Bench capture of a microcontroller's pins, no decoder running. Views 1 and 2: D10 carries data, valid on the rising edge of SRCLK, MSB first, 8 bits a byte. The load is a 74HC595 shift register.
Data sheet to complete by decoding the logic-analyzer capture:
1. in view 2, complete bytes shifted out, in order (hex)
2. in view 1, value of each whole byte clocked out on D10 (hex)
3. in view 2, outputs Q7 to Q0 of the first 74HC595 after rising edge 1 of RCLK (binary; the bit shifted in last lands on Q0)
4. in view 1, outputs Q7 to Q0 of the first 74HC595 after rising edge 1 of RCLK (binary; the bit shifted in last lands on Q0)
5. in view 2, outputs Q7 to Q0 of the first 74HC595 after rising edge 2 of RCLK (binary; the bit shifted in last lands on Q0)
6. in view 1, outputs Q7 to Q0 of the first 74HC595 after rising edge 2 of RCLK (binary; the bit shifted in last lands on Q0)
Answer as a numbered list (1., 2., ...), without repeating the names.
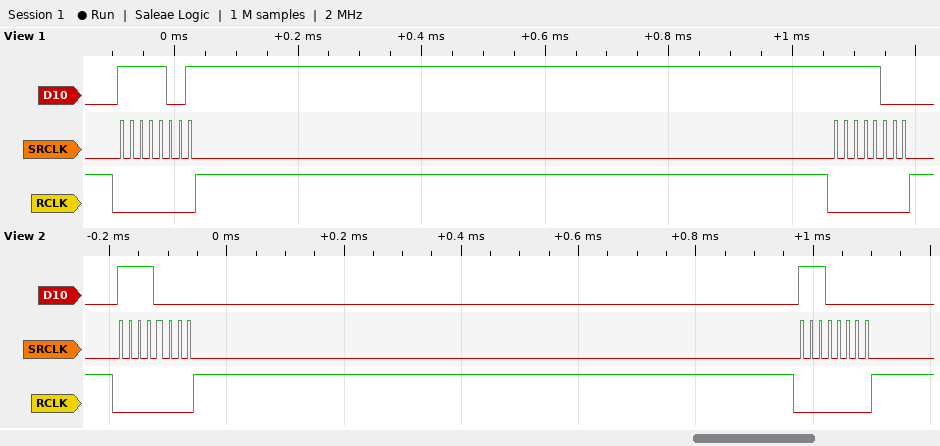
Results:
1. F0 E0
2. 0xF9 0xF8
3. 11110000
4. 11111001
5. 11100000
6. 11111000
